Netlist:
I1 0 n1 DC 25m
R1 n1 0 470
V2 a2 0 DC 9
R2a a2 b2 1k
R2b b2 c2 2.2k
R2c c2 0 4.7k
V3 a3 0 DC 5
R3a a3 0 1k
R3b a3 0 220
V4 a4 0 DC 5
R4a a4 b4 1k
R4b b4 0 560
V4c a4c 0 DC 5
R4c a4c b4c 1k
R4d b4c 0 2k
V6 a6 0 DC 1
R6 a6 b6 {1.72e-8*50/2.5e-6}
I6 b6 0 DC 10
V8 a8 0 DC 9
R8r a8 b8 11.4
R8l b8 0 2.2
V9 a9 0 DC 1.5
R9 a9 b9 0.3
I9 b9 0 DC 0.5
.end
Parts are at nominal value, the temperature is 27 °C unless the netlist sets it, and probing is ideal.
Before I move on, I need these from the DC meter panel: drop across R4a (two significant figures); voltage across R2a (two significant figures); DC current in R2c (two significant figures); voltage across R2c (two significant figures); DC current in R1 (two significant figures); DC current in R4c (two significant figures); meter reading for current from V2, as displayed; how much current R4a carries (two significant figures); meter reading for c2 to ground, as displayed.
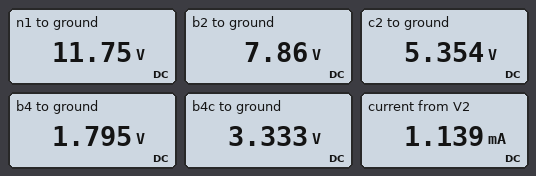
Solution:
3.2 V
1.1 V
1.1 mA
5.4 V
25 mA
1.7 mA
1.139 mA
3.2 mA
5.354 V
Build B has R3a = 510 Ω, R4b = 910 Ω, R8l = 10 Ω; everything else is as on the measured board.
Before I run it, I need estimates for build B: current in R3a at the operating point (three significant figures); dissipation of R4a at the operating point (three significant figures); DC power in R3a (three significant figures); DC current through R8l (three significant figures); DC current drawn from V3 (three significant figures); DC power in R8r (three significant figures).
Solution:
9.80 mA
6.85 mW
49.0 mW
421 mA
32.5 mA
2.02 W
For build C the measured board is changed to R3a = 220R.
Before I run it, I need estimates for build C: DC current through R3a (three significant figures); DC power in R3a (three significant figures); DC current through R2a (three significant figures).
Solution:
22.7 mA
114 mW
1.14 mA
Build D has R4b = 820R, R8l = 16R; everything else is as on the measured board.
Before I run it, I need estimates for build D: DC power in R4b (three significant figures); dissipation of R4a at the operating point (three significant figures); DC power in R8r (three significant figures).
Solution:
6.19 mW
7.55 mW
1.23 W
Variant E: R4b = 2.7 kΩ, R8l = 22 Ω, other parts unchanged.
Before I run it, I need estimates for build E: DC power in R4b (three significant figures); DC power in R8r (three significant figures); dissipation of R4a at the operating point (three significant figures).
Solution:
4.93 mW
828 mW
1.83 mW
